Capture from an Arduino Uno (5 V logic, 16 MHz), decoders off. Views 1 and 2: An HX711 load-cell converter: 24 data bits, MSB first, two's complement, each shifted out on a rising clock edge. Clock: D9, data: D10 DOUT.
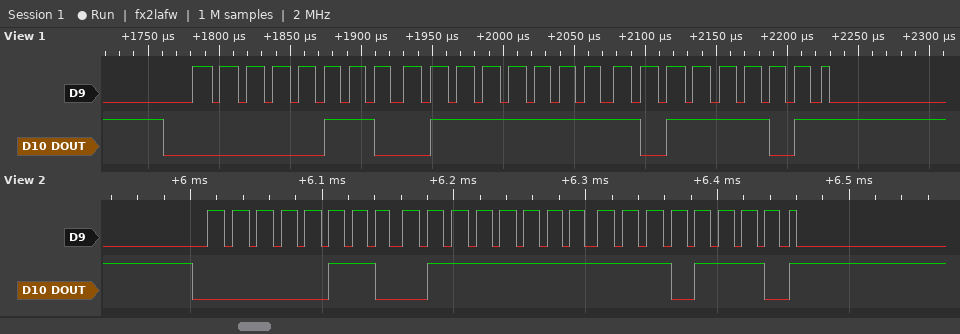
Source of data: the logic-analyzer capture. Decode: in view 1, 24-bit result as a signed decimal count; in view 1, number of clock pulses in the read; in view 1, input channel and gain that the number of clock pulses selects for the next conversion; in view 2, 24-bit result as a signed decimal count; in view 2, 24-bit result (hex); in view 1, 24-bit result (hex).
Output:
425917
25
channel A, gain 128
425966
0x067FEE
0x067FBD
